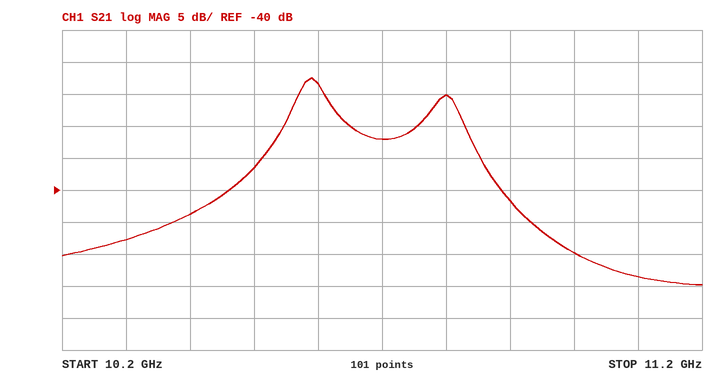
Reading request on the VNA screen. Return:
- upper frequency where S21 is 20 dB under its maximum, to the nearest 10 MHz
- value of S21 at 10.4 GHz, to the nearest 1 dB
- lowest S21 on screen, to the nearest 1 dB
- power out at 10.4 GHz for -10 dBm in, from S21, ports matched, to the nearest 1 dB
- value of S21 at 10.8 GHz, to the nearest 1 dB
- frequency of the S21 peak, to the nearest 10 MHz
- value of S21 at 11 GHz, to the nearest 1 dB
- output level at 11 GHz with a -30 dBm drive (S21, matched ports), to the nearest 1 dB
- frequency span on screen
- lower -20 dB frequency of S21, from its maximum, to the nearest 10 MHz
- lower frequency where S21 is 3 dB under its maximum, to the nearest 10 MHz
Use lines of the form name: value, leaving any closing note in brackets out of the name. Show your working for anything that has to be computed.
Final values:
upper frequency where S21 is 20 dB under its maximum, to the nearest 10 MHz: 10.91 GHz
value of S21 at 10.4 GHz, to the nearest 1 dB: -44 dB
lowest S21 on screen, to the nearest 1 dB: -55 dB
power out at 10.4 GHz for -10 dBm in, from S21, ports matched, to the nearest 1 dB: -10 dBm + (-44 dB) = -54 dBm
value of S21 at 10.8 GHz, to the nearest 1 dB: -25 dB
frequency of the S21 peak, to the nearest 10 MHz: 10.59 GHz
value of S21 at 11 GHz, to the nearest 1 dB: -50 dB
output level at 11 GHz with a -30 dBm drive (S21, matched ports), to the nearest 1 dB: -30 dBm + (-50 dB) = -80 dBm
frequency span on screen: 1 GHz
lower -20 dB frequency of S21, from its maximum, to the nearest 10 MHz: 10.42 GHz
lower frequency where S21 is 3 dB under its maximum, to the nearest 10 MHz: 10.57 GHz
